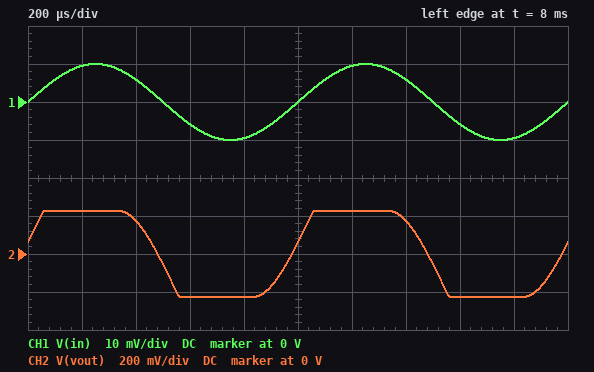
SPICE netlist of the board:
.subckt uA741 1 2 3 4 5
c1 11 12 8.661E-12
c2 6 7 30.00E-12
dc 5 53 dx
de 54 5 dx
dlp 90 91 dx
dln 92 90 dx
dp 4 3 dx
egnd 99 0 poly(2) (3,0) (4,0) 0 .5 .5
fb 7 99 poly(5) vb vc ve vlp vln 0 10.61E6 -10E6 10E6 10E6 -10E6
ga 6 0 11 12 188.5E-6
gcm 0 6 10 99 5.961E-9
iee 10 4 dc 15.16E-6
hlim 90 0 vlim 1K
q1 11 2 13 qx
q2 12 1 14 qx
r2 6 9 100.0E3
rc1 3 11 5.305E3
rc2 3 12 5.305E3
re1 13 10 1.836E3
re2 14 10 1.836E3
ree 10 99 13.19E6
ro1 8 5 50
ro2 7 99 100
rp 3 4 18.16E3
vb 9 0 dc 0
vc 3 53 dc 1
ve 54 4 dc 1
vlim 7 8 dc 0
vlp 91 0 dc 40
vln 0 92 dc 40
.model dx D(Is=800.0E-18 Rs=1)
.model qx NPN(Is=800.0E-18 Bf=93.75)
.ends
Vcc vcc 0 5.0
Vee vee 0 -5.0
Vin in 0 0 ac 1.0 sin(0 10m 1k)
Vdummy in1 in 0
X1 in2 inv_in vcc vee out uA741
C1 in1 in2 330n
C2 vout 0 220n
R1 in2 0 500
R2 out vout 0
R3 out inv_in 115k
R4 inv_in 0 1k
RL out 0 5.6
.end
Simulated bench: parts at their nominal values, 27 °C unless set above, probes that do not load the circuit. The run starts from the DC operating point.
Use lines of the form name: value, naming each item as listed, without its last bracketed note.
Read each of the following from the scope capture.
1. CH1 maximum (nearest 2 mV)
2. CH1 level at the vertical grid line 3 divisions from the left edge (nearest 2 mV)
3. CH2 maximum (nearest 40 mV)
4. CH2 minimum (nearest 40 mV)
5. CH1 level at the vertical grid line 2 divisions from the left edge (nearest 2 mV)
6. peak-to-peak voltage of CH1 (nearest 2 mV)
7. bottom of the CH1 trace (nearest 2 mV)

CH1 maximum: 10 mV
CH1 level at the vertical grid line 3 divisions from the left edge: -6 mV
CH2 maximum: 240 mV
CH2 minimum: -240 mV
CH1 level at the vertical grid line 2 divisions from the left edge: 6 mV
peak-to-peak voltage of CH1: 20 mV
bottom of the CH1 trace: -10 mV
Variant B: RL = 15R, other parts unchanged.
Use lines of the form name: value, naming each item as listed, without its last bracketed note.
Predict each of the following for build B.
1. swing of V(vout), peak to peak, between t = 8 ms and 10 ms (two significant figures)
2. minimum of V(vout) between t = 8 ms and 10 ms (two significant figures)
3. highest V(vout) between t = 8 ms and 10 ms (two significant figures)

swing of V(vout), peak to peak, between t = 8 ms and 10 ms: 1.2 V
minimum of V(vout) between t = 8 ms and 10 ms: -610 mV
highest V(vout) between t = 8 ms and 10 ms: 610 mV
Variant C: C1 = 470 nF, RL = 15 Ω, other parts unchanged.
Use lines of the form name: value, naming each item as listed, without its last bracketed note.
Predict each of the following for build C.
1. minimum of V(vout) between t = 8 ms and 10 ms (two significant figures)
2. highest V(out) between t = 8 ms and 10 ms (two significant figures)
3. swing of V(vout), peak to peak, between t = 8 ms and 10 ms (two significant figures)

minimum of V(vout) between t = 8 ms and 10 ms: -610 mV
highest V(out) between t = 8 ms and 10 ms: 610 mV
swing of V(vout), peak to peak, between t = 8 ms and 10 ms: 1.2 V
